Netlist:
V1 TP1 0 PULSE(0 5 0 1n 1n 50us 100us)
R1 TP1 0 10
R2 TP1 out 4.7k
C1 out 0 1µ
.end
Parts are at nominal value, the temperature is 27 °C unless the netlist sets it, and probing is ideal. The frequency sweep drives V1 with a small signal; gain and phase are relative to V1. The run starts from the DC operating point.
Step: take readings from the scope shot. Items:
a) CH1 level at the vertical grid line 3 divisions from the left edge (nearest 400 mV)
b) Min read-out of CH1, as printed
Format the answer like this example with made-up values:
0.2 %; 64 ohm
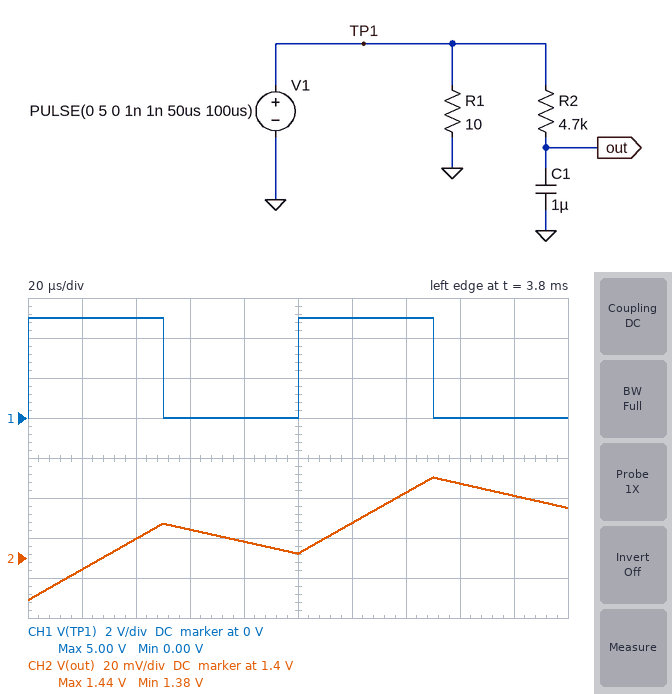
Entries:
0 V; 0.00 V
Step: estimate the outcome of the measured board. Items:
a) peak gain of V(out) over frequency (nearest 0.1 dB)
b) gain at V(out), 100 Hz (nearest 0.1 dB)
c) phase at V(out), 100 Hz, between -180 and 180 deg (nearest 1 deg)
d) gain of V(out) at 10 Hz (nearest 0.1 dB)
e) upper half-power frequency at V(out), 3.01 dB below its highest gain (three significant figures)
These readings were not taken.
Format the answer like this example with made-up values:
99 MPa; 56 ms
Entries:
0 dB; -9.9 dB; -71 deg; -0.4 dB; 33.9 Hz
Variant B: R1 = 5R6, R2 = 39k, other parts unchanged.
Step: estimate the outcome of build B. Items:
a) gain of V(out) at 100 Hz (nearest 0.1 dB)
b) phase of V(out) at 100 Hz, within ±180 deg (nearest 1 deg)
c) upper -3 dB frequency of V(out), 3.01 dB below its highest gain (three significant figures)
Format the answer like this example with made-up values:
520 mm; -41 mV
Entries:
-27.8 dB; -88 deg; 4.08 Hz
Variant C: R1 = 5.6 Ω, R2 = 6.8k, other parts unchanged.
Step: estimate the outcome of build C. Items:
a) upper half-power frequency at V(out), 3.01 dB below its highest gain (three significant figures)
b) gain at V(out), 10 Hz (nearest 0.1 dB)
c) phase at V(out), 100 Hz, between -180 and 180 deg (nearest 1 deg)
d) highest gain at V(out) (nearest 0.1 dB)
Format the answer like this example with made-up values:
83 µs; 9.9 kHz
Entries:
23.4 Hz; -0.7 dB; -77 deg; 0 dB
